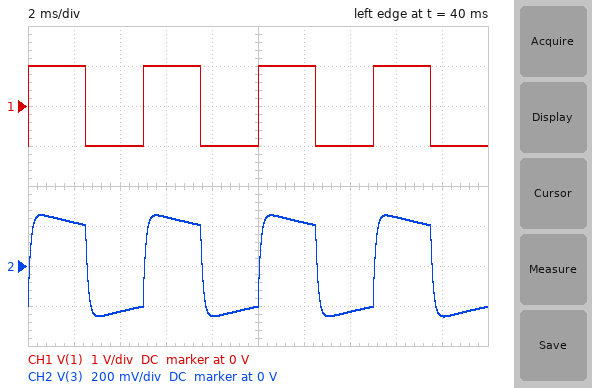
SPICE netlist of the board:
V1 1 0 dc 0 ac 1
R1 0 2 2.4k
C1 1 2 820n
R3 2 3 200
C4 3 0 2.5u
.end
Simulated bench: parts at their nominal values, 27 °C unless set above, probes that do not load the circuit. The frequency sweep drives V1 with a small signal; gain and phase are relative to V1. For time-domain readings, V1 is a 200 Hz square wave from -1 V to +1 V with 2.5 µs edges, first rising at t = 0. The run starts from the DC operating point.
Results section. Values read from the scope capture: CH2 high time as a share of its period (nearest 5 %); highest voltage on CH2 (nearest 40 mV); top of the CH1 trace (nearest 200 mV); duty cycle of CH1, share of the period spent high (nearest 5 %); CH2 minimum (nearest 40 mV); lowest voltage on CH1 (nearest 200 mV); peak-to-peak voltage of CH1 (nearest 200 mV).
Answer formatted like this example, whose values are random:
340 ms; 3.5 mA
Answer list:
50 %; 240 mV; 1.0 V; 50 %; -240 mV; -1.0 V; 2.0 V
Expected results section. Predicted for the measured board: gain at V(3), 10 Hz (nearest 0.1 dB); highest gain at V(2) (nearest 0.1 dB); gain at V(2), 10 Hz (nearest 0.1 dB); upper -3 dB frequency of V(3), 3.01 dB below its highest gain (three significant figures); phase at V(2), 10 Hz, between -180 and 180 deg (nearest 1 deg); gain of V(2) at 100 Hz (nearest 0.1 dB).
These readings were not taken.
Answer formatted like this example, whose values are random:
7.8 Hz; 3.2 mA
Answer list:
-19.2 dB; 0 dB; -19.2 dB; 1.39 kHz; 64 deg; -12.3 dB
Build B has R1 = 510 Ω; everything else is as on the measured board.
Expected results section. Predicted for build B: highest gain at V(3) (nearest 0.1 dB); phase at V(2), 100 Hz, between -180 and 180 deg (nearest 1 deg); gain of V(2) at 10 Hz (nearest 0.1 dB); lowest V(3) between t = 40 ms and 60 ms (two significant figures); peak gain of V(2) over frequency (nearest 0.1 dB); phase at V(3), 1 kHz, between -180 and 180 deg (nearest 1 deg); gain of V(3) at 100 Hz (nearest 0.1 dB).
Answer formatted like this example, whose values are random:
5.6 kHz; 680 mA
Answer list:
-14.4 dB; 51 deg; -31.7 dB; -260 mV; 0 dB; -28 deg; -16.0 dB
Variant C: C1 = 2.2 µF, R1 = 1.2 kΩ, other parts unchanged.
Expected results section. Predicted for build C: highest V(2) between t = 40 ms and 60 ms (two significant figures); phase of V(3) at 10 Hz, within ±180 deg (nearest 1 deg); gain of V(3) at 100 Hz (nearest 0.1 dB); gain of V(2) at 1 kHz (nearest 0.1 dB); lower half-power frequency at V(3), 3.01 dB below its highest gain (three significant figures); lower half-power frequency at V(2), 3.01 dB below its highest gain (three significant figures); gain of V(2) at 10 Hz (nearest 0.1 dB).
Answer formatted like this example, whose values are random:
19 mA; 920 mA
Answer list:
1.7 V; 69 deg; -7.4 dB; -1.4 dB; 25.1 Hz; 555 Hz; -16.2 dB
